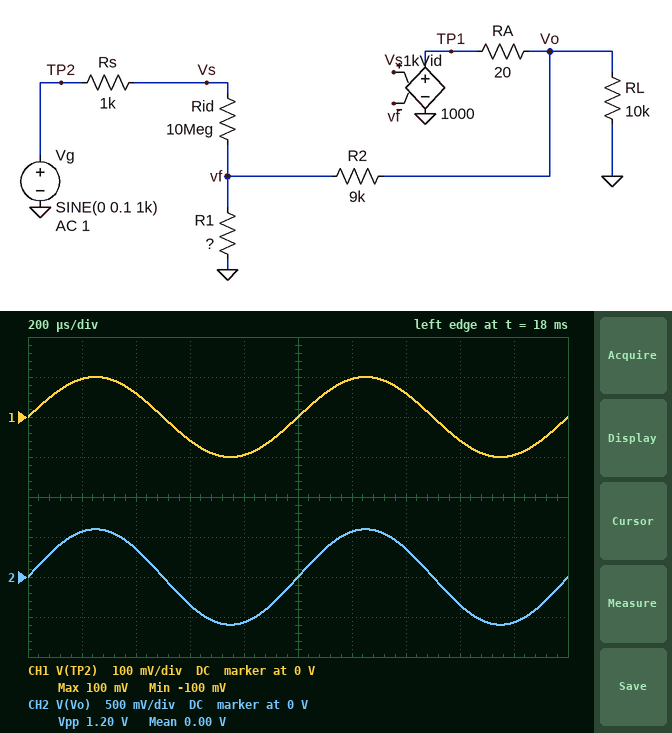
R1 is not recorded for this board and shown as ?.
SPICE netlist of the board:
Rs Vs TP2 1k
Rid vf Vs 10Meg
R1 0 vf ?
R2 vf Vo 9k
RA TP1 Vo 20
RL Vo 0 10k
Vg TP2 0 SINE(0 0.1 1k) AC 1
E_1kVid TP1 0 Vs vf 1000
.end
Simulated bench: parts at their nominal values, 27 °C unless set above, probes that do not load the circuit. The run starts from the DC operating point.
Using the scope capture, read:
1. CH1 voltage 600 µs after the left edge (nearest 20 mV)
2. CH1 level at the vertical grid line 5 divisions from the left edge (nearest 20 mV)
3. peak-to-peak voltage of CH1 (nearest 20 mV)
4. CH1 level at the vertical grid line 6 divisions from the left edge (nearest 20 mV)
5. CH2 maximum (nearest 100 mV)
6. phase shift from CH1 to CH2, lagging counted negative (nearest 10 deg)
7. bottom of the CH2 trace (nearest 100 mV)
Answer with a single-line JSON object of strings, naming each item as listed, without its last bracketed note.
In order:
{"CH1 voltage 600 µs after the left edge": "-60 mV", "CH1 level at the vertical grid line 5 divisions from the left edge": "0 V", "peak-to-peak voltage of CH1": "200 mV", "CH1 level at the vertical grid line 6 divisions from the left edge": "100 mV", "CH2 maximum": "600 mV", "phase shift from CH1 to CH2, lagging counted negative": "0 deg", "bottom of the CH2 trace": "-600 mV"}
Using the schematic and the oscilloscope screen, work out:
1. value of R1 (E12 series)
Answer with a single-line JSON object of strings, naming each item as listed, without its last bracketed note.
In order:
{"value of R1": "1.8 kΩ"}
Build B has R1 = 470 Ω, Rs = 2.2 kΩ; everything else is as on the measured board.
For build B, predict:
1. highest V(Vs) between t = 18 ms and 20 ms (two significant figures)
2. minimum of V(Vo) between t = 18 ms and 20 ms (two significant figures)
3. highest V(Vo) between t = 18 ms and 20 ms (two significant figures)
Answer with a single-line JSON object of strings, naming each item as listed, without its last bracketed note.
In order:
{"highest V(Vs) between t = 18 ms and 20 ms": "100 mV", "minimum of V(Vo) between t = 18 ms and 20 ms": "-2.0 V", "highest V(Vo) between t = 18 ms and 20 ms": "2.0 V"}
